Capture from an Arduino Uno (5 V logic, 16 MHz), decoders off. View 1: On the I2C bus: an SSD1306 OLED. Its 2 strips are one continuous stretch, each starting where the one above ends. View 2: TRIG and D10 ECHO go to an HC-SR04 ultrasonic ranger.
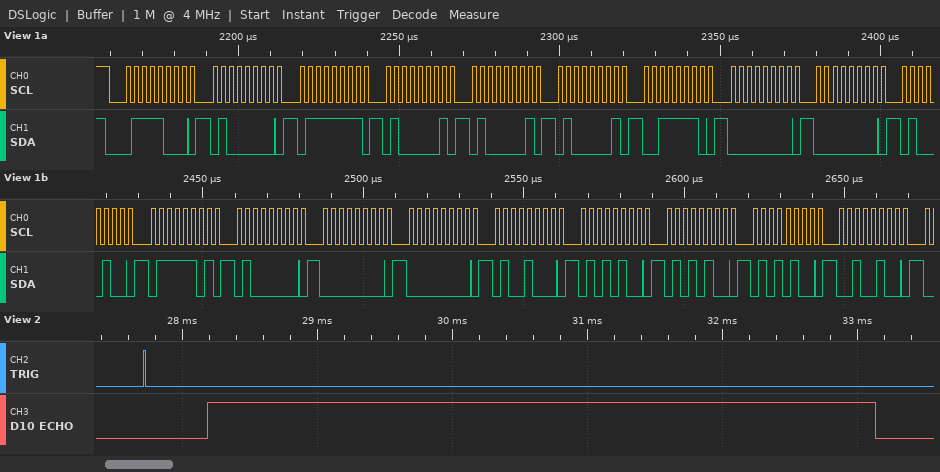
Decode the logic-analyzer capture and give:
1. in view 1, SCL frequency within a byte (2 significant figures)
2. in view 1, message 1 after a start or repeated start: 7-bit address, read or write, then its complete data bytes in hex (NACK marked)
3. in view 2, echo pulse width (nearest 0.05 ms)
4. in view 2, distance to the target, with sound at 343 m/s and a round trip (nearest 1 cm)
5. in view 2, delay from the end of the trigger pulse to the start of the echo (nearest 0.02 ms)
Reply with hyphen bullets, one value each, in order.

- 400 kHz
- 0x3C write: 40 7F 41 41 41 3E 00 00 44 7D 40 00 00 48 54 54 54 24
- 4.95 ms
- 85 cm
- 0.46 ms
